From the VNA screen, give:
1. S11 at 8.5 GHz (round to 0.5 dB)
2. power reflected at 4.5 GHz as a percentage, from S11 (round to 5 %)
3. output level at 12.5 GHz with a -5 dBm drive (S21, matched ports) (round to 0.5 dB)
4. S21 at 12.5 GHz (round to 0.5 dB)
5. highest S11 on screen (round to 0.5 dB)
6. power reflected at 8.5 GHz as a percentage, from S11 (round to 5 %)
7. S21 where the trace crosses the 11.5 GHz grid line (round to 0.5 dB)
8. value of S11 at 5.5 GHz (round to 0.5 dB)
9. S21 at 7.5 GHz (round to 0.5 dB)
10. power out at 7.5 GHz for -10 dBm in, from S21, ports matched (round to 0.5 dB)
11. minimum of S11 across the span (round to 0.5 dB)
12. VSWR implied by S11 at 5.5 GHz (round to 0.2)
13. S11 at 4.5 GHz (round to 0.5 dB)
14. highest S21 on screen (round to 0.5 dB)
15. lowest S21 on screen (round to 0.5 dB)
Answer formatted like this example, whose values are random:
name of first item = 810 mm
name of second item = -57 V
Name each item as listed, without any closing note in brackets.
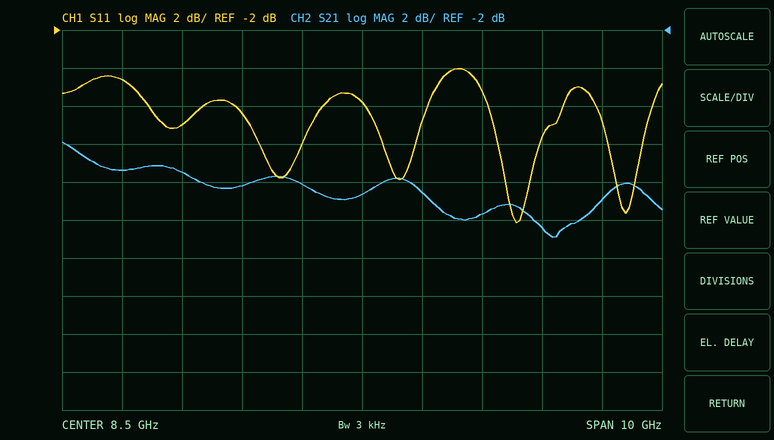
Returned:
S11 at 8.5 GHz = -6.0 dB
power reflected at 4.5 GHz as a percentage, from S11 = 35 %
output level at 12.5 GHz with a -5 dBm drive (S21, matched ports) = -16.0 dBm
S21 at 12.5 GHz = -11.0 dB
highest S11 on screen = -4.0 dB
power reflected at 8.5 GHz as a percentage, from S11 = 25 %
S21 where the trace crosses the 11.5 GHz grid line = -12.5 dB
value of S11 at 5.5 GHz = -7.0 dB
S21 at 7.5 GHz = -10.0 dB
power out at 7.5 GHz for -10 dBm in, from S21, ports matched = -20.0 dBm
minimum of S11 across the span = -12.0 dB
VSWR implied by S11 at 5.5 GHz = 2.6
S11 at 4.5 GHz = -4.5 dB
highest S21 on screen = -8.0 dB
lowest S21 on screen = -13.0 dB
